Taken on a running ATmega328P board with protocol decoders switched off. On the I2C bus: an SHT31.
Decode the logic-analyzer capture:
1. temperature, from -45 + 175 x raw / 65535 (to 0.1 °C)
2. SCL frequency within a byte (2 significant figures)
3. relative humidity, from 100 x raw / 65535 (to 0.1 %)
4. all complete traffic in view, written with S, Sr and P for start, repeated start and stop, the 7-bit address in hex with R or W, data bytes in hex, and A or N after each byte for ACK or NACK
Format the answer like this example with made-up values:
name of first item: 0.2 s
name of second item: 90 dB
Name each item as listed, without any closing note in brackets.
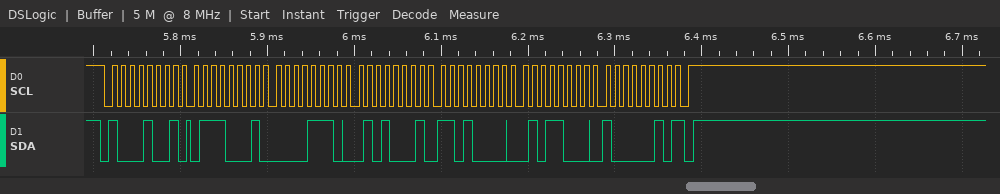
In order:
temperature, from -45 + 175 x raw / 65535: 32.3 °C
SCL frequency within a byte: 100 kHz
relative humidity, from 100 x raw / 65535: 81.4 %
all complete traffic in view, written with S, Sr and P for start, repeated start and stop, the 7-bit address in hex with R or W, data bytes in hex, and A or N after each byte for ACK or NACK: S 44R A 71 A 0E A 51 A D0 A 58 A 82 N P
